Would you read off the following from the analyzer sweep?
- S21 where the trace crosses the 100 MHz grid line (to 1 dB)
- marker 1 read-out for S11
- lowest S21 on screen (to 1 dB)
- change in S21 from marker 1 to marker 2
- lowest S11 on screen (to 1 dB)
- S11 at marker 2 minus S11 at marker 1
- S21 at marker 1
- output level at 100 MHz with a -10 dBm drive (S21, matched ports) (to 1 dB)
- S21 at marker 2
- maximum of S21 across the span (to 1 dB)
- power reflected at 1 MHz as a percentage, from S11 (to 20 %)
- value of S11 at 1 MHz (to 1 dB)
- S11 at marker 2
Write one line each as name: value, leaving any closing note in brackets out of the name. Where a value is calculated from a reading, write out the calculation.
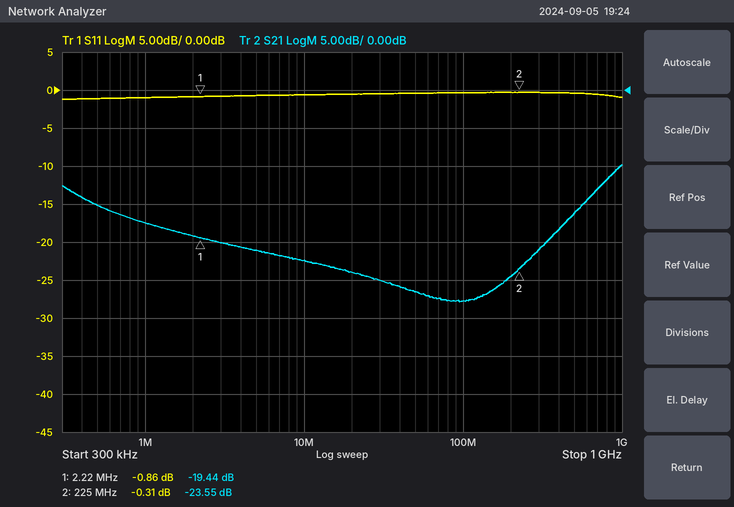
S21 where the trace crosses the 100 MHz grid line: -28 dB
marker 1 read-out for S11: -0.86 dB
lowest S21 on screen: -28 dB
change in S21 from marker 1 to marker 2: -23.55 − (-19.44) = -4.11 dB
lowest S11 on screen: -1 dB
S11 at marker 2 minus S11 at marker 1: -0.31 − (-0.86) = 0.55 dB
S21 at marker 1: -19.44 dB
output level at 100 MHz with a -10 dBm drive (S21, matched ports): -10 dBm + (-28 dB) = -38 dBm
S21 at marker 2: -23.55 dB
maximum of S21 across the span: -10 dB
power reflected at 1 MHz as a percentage, from S11: 10^(-1/10) ≈ 79.4 %, so 80 % to the nearest 20 %
value of S11 at 1 MHz: -1 dB
S11 at marker 2: -0.31 dB
